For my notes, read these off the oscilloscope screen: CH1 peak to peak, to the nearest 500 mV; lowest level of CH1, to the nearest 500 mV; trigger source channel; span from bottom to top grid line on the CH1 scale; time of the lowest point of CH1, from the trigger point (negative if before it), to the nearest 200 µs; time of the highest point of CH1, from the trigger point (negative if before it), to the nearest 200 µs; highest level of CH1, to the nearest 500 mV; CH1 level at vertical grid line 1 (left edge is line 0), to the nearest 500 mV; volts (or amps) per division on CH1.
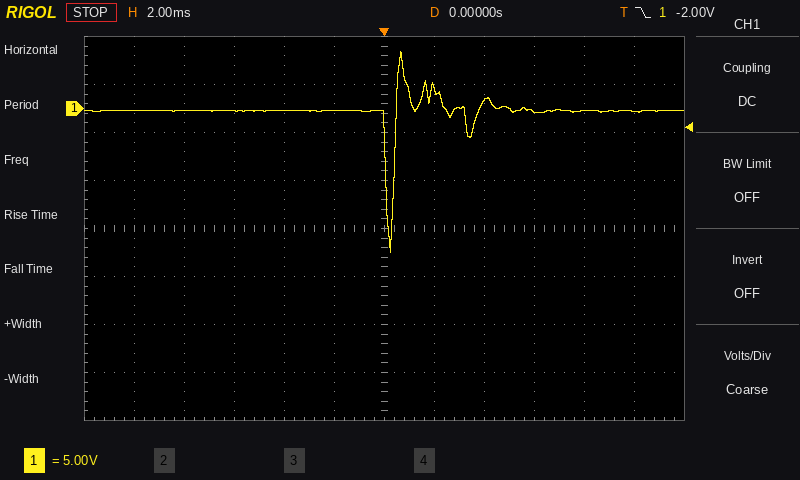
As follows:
21.0 V
-15.0 V
CH1
40 V
+200 µs
+600 µs
6.0 V
0.0 V
5 V
